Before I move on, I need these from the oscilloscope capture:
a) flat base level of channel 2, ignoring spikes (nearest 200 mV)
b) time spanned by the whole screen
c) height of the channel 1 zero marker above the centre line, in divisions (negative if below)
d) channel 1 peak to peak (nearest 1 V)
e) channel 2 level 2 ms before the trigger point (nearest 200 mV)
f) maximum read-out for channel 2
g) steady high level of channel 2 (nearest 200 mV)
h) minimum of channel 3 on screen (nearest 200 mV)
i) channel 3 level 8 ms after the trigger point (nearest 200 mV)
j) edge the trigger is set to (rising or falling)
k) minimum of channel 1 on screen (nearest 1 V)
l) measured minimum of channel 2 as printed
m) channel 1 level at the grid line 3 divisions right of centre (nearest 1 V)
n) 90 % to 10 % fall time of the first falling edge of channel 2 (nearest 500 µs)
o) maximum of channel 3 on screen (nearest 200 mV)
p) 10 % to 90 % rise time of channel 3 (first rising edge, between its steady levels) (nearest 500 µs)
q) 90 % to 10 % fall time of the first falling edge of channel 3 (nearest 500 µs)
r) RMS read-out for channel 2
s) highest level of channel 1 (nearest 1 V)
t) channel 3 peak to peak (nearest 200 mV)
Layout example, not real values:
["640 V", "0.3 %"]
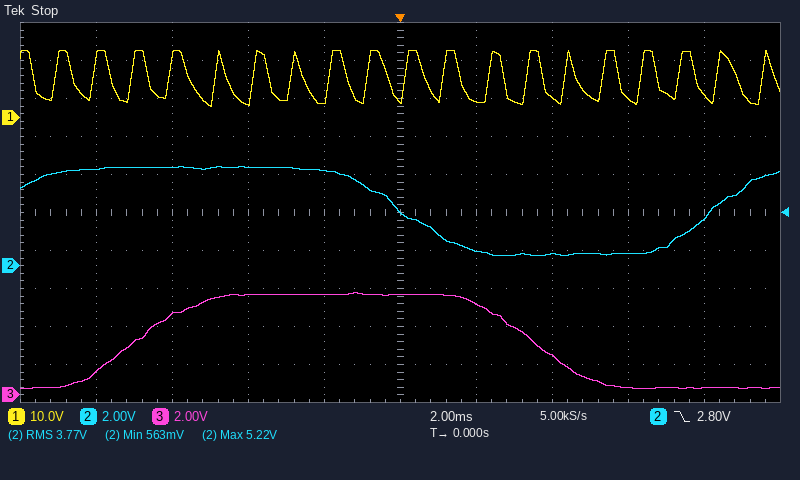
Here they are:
["600 mV", "20 ms", "+2.5 div", "15 V", "5.0 V", "5.22 V", "5.2 V", "400 mV", "400 mV", "falling", "3 V", "563 mV", "5 V", "3.0 ms", "5.4 V", "3.0 ms", "3.0 ms", "3.77 V", "18 V", "5.0 V"]
